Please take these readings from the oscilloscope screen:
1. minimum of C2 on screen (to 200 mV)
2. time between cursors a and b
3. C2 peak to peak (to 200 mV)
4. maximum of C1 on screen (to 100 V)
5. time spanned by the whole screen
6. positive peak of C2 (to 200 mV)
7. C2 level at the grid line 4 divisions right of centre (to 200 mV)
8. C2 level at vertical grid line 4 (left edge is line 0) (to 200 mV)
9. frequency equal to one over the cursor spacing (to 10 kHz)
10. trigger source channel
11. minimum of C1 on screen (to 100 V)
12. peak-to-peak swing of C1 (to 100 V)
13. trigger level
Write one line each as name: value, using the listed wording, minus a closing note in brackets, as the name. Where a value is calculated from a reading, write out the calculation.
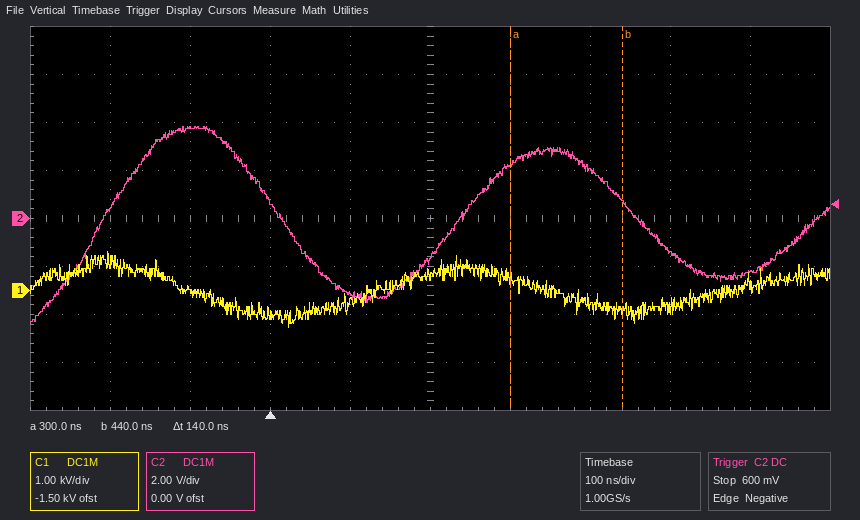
minimum of C2 on screen: -4.4 V
time between cursors a and b: 140 ns
C2 peak to peak: 3.8 V − (-4.4 V) = 8.2 V
maximum of C1 on screen: 800 V
time spanned by the whole screen: 1 µs
positive peak of C2: 3.8 V
C2 level at the grid line 4 divisions right of centre: -2.2 V
C2 level at vertical grid line 4 (left edge is line 0): -3.2 V
frequency equal to one over the cursor spacing: 1 / 140 ns ≈ 7.14 MHz
trigger source channel: C2
minimum of C1 on screen: -800 V
peak-to-peak swing of C1: 800 V − (-800 V) = 1.6 kV
trigger level: 600 mV
